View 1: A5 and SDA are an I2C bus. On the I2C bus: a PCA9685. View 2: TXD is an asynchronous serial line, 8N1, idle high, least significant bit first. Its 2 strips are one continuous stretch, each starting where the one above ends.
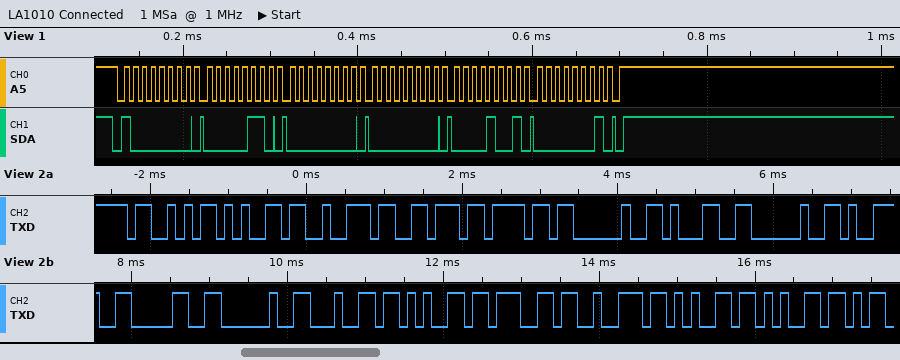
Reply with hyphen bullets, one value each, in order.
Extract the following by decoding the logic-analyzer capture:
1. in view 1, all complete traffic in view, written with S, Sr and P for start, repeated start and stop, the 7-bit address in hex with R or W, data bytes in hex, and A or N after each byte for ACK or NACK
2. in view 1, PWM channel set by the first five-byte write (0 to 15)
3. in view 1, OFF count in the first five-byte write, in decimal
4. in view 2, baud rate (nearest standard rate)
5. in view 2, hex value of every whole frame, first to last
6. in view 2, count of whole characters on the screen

- S 40W A 06 A 00 A 00 A 09 A 01 A P
- 0
- 265
- 9600 baud
- 53 65 72 76 6F 20 31 20 39 30 20 64 65 67 72 65 65
- 17
